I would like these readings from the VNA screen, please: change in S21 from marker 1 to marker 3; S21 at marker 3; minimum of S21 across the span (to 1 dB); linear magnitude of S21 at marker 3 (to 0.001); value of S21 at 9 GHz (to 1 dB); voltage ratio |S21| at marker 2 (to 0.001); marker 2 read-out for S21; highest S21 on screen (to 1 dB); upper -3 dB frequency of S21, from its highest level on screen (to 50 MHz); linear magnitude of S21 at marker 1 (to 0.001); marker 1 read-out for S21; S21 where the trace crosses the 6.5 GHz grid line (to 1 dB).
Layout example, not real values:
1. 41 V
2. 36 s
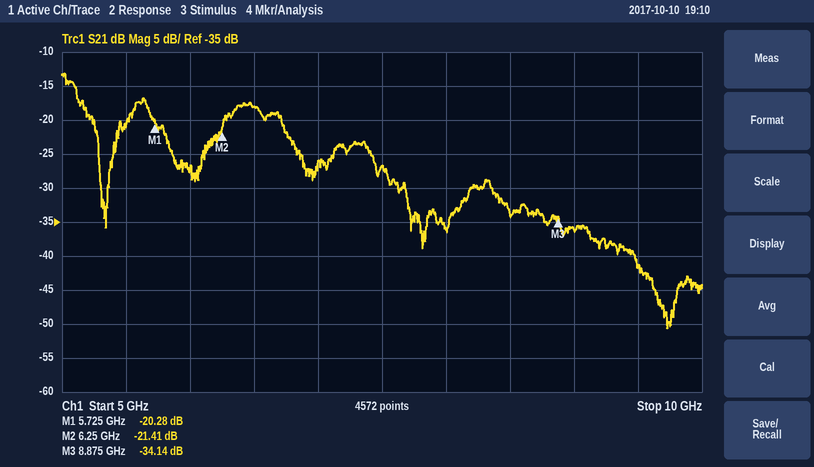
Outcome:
1. -13.86 dB
2. -34.14 dB
3. -51 dB
4. 0.020
5. -36 dB
6. 0.085
7. -21.41 dB
8. -13 dB
9. 5.10 GHz
10. 0.097
11. -20.28 dB
12. -18 dB
